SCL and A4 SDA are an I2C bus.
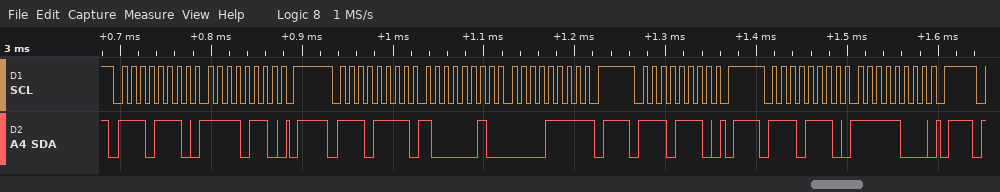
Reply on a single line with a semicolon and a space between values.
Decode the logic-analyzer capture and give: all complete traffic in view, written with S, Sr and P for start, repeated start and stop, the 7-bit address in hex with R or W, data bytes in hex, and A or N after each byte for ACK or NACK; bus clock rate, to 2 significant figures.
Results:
S 77W A F6 A P S 77R A 82 A 0F N P S 77W A P S 77W A F8 A P; 100 kHz
